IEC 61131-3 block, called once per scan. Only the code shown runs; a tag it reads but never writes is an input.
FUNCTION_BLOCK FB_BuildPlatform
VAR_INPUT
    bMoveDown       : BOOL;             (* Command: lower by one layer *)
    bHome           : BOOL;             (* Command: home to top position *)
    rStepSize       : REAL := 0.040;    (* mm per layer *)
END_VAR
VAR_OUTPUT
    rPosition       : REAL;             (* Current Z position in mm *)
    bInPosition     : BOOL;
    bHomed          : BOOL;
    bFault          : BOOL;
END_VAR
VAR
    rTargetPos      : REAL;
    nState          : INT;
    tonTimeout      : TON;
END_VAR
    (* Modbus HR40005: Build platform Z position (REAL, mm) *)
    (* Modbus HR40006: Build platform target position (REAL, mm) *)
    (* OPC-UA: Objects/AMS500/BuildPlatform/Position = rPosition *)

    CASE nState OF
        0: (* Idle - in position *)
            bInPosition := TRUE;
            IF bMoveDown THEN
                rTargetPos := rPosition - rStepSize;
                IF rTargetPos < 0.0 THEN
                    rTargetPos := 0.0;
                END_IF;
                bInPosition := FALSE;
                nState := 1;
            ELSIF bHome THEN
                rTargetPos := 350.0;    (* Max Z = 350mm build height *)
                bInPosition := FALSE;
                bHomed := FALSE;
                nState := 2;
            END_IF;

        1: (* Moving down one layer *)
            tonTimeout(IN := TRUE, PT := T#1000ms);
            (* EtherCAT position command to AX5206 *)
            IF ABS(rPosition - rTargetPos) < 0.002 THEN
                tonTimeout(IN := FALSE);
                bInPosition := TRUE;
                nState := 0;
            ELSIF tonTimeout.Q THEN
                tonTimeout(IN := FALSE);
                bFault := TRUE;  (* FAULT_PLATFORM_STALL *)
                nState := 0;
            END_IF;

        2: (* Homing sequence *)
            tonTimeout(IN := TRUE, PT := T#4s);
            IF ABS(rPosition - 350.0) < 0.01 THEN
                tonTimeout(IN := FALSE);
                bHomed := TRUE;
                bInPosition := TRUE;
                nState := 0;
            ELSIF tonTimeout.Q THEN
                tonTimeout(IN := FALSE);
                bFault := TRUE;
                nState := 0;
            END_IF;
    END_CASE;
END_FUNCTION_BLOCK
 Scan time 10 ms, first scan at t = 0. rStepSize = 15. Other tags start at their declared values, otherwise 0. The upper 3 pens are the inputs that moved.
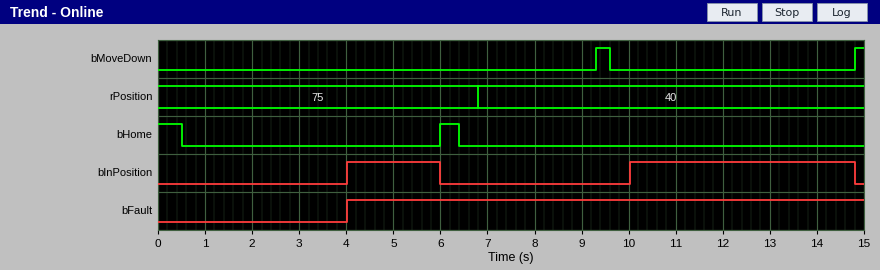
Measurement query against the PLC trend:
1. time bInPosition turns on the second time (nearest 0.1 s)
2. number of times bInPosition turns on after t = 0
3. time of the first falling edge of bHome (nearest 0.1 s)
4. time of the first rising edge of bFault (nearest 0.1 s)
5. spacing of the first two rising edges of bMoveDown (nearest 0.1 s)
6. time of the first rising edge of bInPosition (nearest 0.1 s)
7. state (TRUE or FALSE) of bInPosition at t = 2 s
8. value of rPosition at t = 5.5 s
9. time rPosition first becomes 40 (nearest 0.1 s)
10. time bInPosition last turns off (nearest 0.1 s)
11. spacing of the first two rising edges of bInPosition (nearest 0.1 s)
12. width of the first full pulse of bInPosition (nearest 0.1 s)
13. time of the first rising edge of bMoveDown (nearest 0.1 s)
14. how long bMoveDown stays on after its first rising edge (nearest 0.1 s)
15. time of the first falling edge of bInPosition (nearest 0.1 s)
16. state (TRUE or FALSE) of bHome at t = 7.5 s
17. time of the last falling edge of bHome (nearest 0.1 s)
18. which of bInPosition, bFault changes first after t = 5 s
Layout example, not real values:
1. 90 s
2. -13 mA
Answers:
1. 10.0 s
2. 2
3. 0.5 s
4. 4.0 s
5. 5.5 s
6. 4.0 s
7. FALSE
8. 75
9. 6.8 s
10. 14.8 s
11. 6.0 s
12. 2.0 s
13. 9.3 s
14. 0.3 s
15. 6.0 s
16. FALSE
17. 6.4 s
18. bInPosition
